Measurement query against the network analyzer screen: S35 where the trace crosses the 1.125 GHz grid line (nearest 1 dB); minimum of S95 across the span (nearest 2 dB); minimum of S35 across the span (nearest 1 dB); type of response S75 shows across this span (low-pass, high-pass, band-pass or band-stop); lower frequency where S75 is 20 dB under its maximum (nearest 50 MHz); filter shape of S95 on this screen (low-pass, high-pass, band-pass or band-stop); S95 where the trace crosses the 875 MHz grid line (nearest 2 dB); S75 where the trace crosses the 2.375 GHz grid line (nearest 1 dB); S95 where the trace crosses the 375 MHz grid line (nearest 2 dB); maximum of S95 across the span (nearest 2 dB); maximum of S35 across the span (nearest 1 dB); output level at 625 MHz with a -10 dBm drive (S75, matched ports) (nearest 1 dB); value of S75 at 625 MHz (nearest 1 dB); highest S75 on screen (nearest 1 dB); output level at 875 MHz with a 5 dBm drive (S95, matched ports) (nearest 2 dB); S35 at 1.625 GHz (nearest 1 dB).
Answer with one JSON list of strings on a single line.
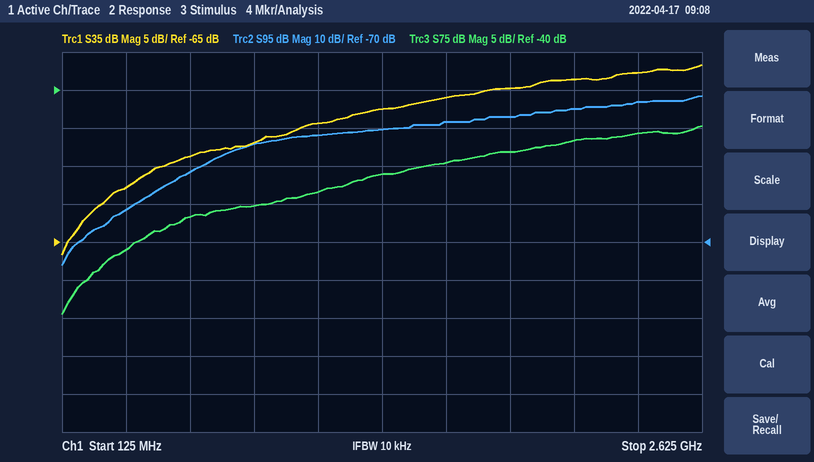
["-49 dB", "-76 dB", "-67 dB", "high-pass", "250 MHz", "high-pass", "-44 dB", "-46 dB", "-62 dB", "-32 dB", "-42 dB", "-67 dBm", "-57 dB", "-45 dB", "-40 dBm", "-46 dB"]
